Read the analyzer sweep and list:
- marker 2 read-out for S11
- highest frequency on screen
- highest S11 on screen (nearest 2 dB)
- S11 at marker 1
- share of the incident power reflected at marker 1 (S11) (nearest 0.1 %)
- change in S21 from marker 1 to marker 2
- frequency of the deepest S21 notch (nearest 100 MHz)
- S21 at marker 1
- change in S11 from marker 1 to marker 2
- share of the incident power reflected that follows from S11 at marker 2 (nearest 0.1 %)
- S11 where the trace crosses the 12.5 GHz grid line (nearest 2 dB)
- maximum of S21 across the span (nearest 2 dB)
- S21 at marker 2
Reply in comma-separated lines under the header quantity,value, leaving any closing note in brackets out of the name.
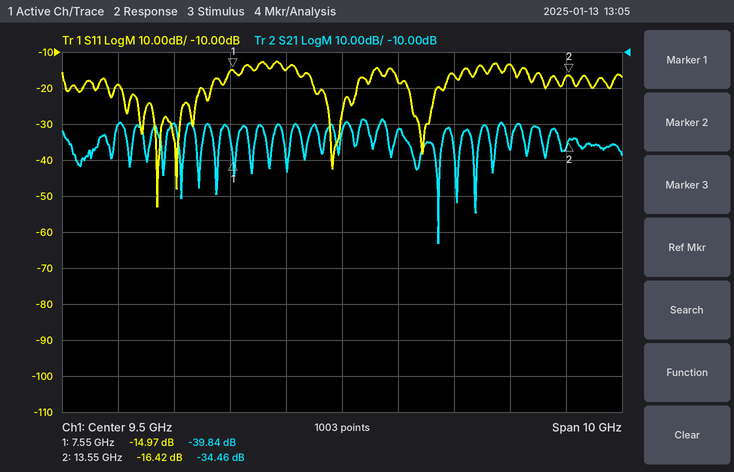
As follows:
quantity,value
marker 2 read-out for S11,-16.42 dB
highest frequency on screen,14.5 GHz
highest S11 on screen,-12 dB
S11 at marker 1,-14.97 dB
share of the incident power reflected at marker 1 (S11),3.2 %
change in S21 from marker 1 to marker 2,5.38 dB
frequency of the deepest S21 notch,11.2 GHz
S21 at marker 1,-39.84 dB
change in S11 from marker 1 to marker 2,-1.45 dB
share of the incident power reflected that follows from S11 at marker 2,2.3 %
S11 where the trace crosses the 12.5 GHz grid line,-14 dB
maximum of S21 across the span,-28 dB
S21 at marker 2,-34.46 dB
